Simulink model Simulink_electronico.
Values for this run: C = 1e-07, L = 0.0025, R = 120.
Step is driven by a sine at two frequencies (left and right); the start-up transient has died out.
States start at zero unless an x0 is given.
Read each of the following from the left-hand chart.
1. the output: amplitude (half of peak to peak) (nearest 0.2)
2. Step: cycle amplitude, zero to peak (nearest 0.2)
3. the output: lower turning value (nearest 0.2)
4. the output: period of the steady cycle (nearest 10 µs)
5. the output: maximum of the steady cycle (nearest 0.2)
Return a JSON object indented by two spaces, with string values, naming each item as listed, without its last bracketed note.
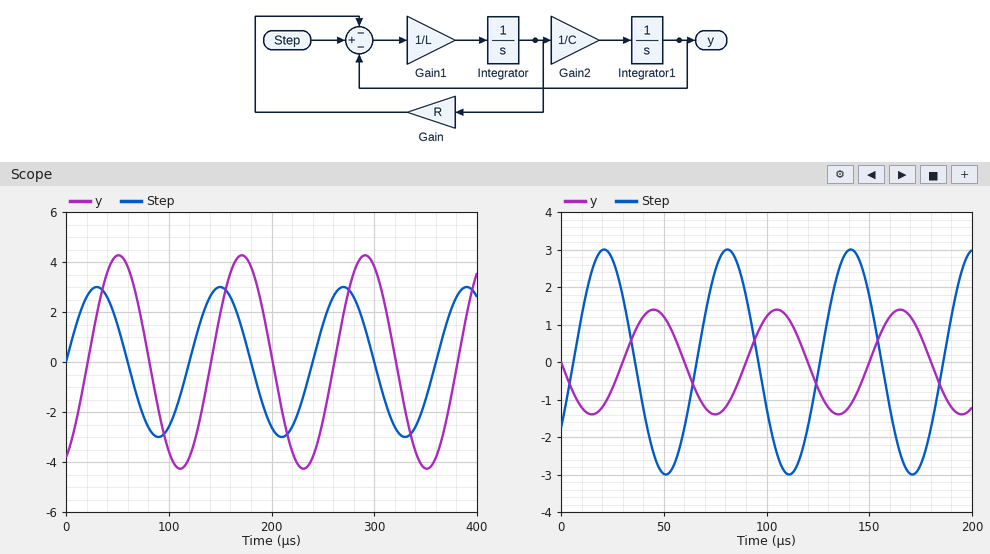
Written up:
{
  "the output: amplitude (half of peak to peak)": "4.2",
  "Step: cycle amplitude, zero to peak": "3.0",
  "the output: lower turning value": "-4.2",
  "the output: period of the steady cycle": "120 µs",
  "the output: maximum of the steady cycle": "4.2"
}
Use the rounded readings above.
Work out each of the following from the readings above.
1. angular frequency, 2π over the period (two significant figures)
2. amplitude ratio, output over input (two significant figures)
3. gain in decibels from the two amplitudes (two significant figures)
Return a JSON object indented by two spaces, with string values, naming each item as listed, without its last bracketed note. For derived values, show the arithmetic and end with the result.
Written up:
{
  "angular frequency, 2π over the period": "2π / 120 = 0.052 rad/µs",
  "amplitude ratio, output over input": "4.2 / 3 = 1.4",
  "gain in decibels from the two amplitudes": "20 log10(4.2 / 3) = 2.9 dB"
}
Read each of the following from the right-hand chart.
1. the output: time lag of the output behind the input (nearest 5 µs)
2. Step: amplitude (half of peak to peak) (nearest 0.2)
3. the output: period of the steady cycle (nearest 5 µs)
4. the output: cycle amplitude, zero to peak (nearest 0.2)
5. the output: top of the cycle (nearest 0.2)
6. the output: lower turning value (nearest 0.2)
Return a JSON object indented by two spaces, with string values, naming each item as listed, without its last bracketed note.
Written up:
{
  "the output: time lag of the output behind the input": "25 µs",
  "Step: amplitude (half of peak to peak)": "3.0",
  "the output: period of the steady cycle": "60 µs",
  "the output: cycle amplitude, zero to peak": "1.4",
  "the output: top of the cycle": "1.4",
  "the output: lower turning value": "-1.4"
}
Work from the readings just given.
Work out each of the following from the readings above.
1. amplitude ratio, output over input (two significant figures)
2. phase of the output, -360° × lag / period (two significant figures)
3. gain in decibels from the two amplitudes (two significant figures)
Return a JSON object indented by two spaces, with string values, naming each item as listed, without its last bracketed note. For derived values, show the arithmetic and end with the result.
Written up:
{
  "amplitude ratio, output over input": "1.4 / 3 = 0.47",
  "phase of the output, -360° × lag / period": "-360 × 25 / 60 = -150°",
  "gain in decibels from the two amplitudes": "20 log10(1.4 / 3) = -6.6 dB"
}
